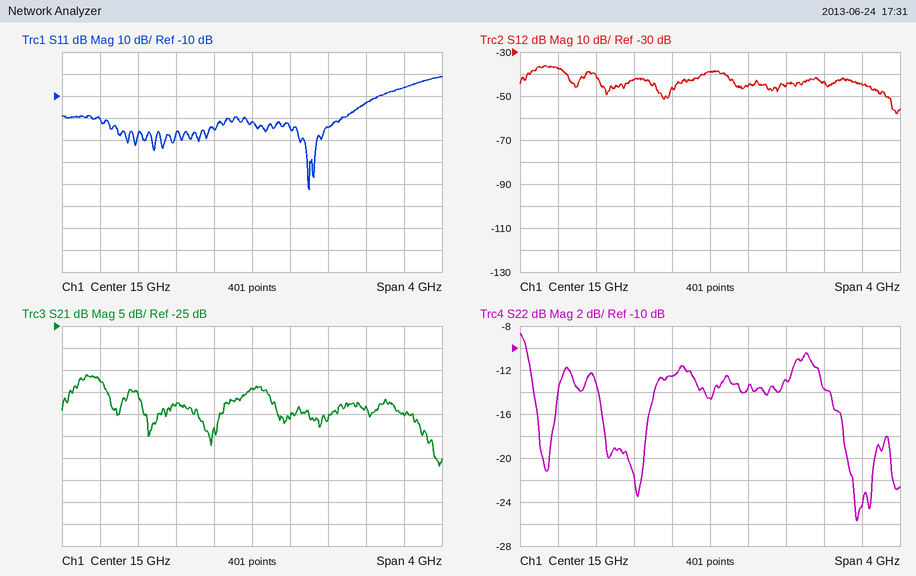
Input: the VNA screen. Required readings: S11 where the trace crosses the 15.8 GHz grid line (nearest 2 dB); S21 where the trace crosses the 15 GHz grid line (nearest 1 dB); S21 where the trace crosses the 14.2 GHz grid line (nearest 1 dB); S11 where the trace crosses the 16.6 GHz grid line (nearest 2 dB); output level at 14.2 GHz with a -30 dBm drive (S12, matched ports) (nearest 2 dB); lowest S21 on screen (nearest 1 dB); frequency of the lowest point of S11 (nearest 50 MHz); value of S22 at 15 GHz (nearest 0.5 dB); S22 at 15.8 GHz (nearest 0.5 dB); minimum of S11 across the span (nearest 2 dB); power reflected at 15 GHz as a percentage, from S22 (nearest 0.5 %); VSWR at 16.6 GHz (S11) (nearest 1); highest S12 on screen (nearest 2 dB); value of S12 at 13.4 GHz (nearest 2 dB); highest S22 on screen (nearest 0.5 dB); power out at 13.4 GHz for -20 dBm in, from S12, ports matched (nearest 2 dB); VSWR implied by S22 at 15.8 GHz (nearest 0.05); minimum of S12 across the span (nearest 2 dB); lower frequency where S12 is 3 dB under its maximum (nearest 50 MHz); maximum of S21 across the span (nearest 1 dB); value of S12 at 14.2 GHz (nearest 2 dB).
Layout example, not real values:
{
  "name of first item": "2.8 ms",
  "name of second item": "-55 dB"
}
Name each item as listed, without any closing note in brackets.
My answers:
{
  "S11 where the trace crosses the 15.8 GHz grid line": "-24 dB",
  "S21 where the trace crosses the 15 GHz grid line": "-39 dB",
  "S21 where the trace crosses the 14.2 GHz grid line": "-43 dB",
  "S11 where the trace crosses the 16.6 GHz grid line": "-6 dB",
  "output level at 14.2 GHz with a -30 dBm drive (S12, matched ports)": "-72 dBm",
  "lowest S21 on screen": "-57 dB",
  "frequency of the lowest point of S11": "15.60 GHz",
  "value of S22 at 15 GHz": "-14.5 dB",
  "S22 at 15.8 GHz": "-13.0 dB",
  "minimum of S11 across the span": "-52 dB",
  "power reflected at 15 GHz as a percentage, from S22": "3.5 %",
  "VSWR at 16.6 GHz (S11)": "3",
  "highest S12 on screen": "-36 dB",
  "value of S12 at 13.4 GHz": "-38 dB",
  "highest S22 on screen": "-8.5 dB",
  "power out at 13.4 GHz for -20 dBm in, from S12, ports matched": "-58 dBm",
  "VSWR implied by S22 at 15.8 GHz": "1.60",
  "minimum of S12 across the span": "-58 dB",
  "lower frequency where S12 is 3 dB under its maximum": "13.10 GHz",
  "maximum of S21 across the span": "-36 dB",
  "value of S12 at 14.2 GHz": "-42 dB"
}
